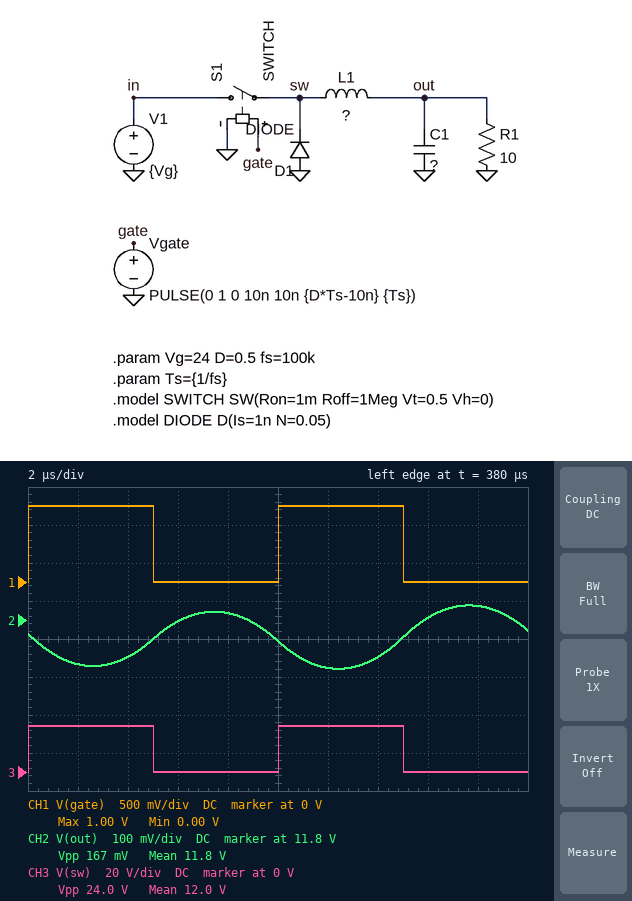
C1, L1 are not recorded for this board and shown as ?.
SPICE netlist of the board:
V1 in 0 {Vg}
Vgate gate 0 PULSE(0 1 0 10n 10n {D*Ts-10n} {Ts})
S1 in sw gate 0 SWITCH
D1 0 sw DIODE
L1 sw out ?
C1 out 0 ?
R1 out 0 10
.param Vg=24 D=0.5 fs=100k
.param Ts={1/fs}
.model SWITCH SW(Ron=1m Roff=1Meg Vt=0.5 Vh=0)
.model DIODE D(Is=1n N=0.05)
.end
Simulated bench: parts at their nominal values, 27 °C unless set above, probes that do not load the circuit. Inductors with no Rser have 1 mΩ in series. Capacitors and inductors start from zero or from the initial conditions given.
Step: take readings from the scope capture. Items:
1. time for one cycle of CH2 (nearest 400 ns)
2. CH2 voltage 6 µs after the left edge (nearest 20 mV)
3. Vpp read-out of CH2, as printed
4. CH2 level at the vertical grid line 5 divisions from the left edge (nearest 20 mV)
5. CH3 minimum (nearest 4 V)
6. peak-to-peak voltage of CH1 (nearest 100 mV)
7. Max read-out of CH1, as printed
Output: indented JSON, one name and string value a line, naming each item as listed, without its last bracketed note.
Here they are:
{
  "time for one cycle of CH2": "10.0 µs",
  "CH2 voltage 6 µs after the left edge": "11.80 V",
  "Vpp read-out of CH2, as printed": "167 mV",
  "CH2 level at the vertical grid line 5 divisions from the left edge": "11.74 V",
  "CH3 minimum": "0 V",
  "peak-to-peak voltage of CH1": "1.0 V",
  "Max read-out of CH1, as printed": "1.00 V"
}
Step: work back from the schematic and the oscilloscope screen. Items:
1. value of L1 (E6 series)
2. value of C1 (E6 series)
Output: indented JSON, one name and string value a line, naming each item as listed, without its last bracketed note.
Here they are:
{
  "value of L1": "33 µH",
  "value of C1": "15 µF"
}
